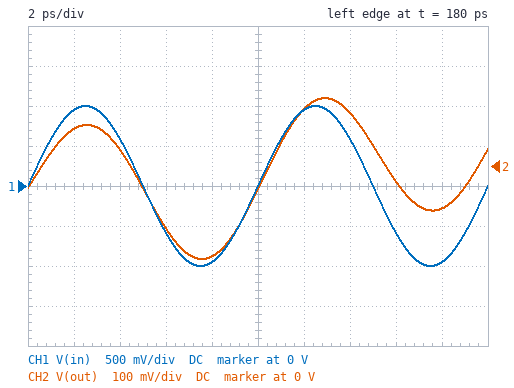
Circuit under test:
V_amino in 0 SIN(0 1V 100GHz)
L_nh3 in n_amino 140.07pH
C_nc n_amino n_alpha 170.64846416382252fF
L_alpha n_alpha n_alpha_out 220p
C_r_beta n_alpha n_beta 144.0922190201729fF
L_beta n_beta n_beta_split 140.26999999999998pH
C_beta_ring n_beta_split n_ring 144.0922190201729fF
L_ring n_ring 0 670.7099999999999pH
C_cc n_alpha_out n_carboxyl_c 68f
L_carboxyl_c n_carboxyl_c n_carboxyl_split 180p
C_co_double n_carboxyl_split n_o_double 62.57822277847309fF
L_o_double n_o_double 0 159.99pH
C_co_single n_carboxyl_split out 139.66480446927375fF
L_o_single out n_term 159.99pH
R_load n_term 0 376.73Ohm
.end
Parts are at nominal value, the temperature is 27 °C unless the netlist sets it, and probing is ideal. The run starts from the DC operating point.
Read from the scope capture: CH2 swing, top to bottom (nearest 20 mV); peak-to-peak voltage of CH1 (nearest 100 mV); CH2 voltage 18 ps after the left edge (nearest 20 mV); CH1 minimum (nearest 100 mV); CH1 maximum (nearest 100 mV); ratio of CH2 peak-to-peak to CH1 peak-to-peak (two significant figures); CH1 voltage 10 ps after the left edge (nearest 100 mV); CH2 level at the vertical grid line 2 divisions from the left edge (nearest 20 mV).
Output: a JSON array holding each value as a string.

["400 mV", "2.0 V", "-100 mV", "-1.0 V", "1.0 V", "0.20", "0 V", "40 mV"]
